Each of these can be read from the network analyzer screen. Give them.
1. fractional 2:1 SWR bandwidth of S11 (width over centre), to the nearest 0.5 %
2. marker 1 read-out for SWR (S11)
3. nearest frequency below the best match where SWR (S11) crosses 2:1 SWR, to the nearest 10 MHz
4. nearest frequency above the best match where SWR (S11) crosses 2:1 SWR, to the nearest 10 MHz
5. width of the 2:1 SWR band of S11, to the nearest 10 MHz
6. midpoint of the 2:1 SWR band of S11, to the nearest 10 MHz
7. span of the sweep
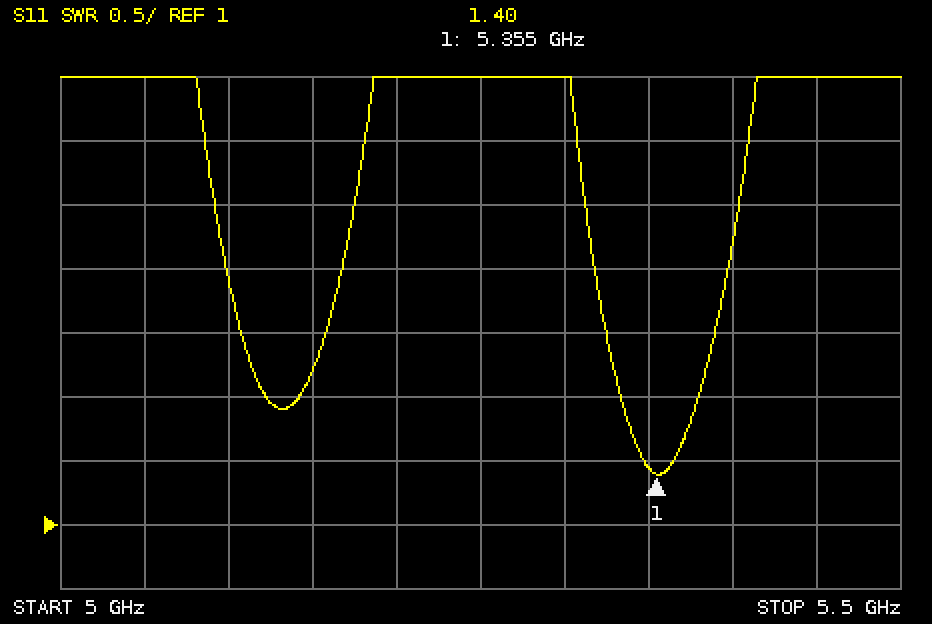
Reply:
1.0 %
1.40
5.33 GHz
5.38 GHz
50 MHz
5.36 GHz
500 MHz
